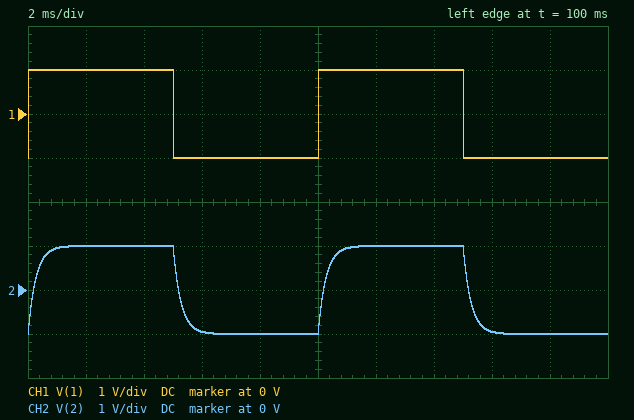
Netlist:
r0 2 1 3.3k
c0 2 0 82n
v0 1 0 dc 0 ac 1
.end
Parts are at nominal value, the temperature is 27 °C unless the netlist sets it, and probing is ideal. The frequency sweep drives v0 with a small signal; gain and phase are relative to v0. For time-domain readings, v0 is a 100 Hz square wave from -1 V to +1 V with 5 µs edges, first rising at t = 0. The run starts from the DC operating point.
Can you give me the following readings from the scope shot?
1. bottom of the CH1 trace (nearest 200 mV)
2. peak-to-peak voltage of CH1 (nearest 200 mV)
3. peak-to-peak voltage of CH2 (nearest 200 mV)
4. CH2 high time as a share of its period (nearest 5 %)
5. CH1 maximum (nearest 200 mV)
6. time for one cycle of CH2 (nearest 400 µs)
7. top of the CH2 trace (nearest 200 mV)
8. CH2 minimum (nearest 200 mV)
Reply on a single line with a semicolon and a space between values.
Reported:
-1.0 V; 2.0 V; 2.0 V; 50 %; 1.0 V; 10.0 ms; 1.0 V; -1.0 V
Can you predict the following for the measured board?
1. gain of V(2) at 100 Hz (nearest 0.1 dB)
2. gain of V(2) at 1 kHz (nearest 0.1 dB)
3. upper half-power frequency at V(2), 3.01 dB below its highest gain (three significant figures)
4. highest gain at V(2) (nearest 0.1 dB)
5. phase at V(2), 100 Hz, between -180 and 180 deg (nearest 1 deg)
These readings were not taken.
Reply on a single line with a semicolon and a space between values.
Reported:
-0.1 dB; -5.9 dB; 588 Hz; 0 dB; -10 deg
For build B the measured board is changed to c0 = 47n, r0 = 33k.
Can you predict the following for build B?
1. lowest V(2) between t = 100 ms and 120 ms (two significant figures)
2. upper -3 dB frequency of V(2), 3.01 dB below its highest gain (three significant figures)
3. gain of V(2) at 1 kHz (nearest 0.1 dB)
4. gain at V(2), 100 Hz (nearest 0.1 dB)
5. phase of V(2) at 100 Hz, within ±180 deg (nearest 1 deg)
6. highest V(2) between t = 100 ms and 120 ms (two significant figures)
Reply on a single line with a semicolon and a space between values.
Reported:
-920 mV; 103 Hz; -19.8 dB; -2.9 dB; -44 deg; 920 mV
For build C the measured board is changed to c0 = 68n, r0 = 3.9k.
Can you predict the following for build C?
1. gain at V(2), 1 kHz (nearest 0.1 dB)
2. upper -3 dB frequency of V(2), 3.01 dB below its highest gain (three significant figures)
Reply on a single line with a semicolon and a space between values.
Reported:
-5.8 dB; 600 Hz
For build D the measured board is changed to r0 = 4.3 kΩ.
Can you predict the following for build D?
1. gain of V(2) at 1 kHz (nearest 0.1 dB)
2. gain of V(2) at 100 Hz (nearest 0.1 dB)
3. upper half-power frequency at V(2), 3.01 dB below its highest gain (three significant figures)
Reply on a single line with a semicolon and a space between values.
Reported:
-7.7 dB; -0.2 dB; 451 Hz
